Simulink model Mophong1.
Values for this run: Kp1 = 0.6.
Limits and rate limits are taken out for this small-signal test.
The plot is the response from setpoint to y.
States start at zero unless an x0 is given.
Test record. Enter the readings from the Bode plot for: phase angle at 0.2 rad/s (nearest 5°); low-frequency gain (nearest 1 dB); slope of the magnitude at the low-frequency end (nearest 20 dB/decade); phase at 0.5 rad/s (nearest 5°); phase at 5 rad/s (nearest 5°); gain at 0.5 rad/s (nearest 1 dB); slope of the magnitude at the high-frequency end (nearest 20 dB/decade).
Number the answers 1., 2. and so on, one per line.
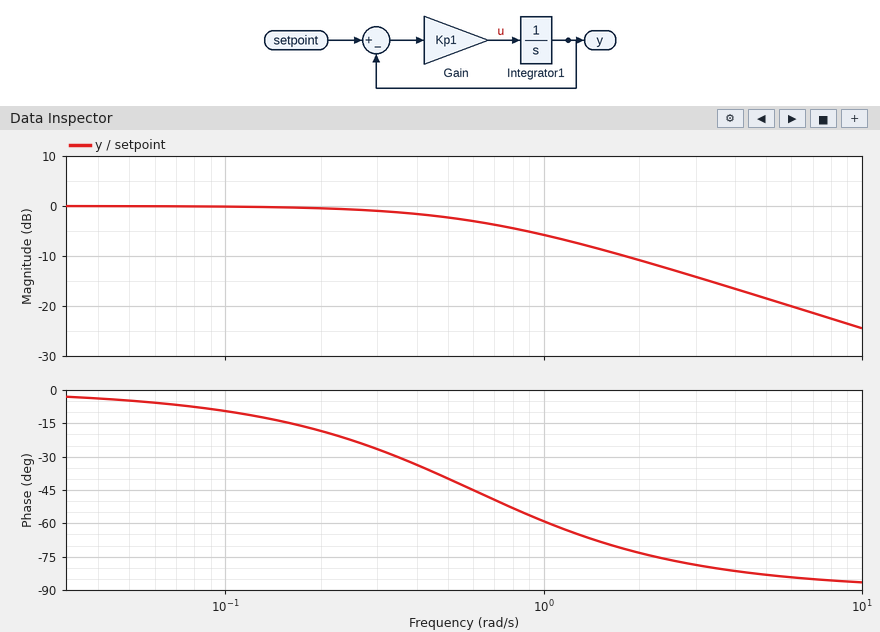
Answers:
1. -20°
2. 0 dB
3. 0 dB/decade
4. -40°
5. -85°
6. -2 dB
7. -20 dB/decade
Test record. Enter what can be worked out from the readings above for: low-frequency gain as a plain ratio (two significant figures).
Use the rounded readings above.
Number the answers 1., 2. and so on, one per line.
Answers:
1. 1.0
